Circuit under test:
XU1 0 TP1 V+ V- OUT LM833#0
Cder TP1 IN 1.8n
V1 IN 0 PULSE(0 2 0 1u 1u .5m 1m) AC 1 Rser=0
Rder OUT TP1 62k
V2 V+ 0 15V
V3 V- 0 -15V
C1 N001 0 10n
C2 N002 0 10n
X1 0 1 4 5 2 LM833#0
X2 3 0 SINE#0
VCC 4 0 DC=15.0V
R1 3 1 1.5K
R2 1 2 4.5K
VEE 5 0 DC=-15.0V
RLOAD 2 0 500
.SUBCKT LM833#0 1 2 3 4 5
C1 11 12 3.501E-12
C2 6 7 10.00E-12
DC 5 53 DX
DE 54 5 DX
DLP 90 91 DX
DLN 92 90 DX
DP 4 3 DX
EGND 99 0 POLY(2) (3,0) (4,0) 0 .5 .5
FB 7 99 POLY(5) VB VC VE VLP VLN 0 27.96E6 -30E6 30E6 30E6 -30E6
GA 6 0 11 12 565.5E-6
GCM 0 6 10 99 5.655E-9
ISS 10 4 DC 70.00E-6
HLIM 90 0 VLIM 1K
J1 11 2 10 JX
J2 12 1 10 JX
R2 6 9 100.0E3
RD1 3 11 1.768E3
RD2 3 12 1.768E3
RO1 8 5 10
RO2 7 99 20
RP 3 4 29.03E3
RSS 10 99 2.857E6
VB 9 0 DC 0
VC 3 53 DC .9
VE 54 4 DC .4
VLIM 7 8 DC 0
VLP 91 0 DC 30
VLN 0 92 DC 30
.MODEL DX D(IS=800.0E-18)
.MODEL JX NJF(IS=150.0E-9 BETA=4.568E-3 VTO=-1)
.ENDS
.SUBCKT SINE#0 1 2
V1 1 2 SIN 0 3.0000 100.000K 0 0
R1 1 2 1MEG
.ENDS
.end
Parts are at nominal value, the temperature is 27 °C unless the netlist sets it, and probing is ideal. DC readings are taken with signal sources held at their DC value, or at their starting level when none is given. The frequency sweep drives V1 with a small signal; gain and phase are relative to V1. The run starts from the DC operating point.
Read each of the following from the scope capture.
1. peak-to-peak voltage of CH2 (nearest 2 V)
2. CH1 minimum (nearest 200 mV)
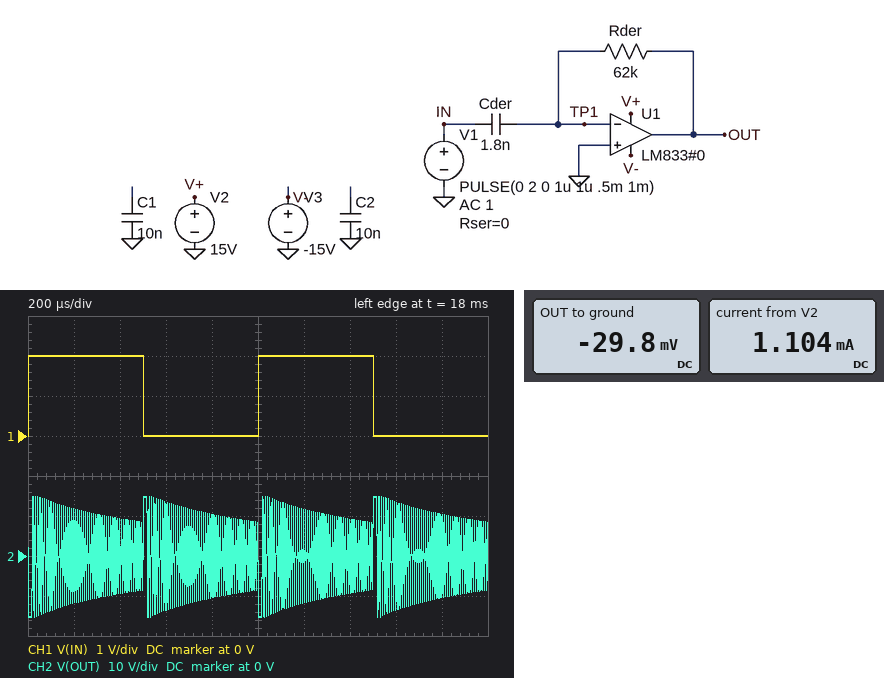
30 V
0 V
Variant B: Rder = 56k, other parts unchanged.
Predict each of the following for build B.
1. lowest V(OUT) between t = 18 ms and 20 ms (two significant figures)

-15 V
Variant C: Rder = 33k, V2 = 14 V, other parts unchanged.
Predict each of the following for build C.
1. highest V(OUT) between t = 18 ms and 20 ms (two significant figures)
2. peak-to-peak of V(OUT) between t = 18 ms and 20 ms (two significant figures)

14 V
29 V
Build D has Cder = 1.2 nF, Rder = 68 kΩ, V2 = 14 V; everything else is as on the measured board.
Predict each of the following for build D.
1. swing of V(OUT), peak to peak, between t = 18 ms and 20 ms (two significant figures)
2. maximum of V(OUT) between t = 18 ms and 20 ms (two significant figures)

29 V
14 V
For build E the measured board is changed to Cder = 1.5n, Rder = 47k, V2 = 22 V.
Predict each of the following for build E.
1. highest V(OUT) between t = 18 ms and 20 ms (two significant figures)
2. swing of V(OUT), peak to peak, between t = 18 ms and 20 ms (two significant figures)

22 V
37 V
